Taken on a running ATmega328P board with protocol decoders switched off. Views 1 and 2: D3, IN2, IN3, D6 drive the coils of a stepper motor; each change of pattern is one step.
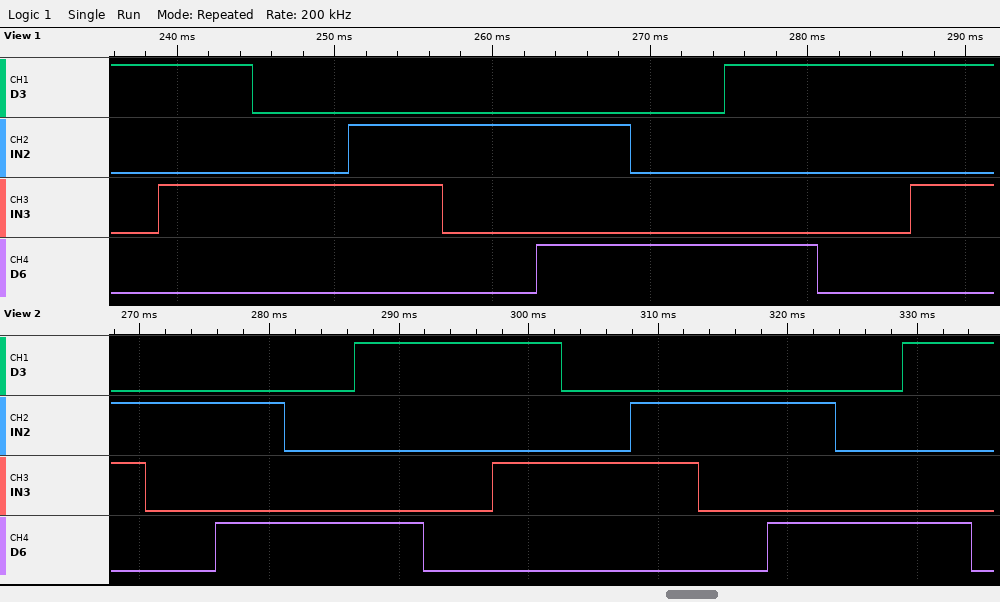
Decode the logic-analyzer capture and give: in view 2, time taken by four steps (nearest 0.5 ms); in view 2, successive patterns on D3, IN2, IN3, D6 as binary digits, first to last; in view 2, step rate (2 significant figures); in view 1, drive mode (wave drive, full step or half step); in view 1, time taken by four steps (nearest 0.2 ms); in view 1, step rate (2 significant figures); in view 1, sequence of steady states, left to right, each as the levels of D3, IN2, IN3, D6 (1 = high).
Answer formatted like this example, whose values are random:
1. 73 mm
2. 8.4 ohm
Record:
1. 21.5 ms
2. 0110 0100 0101 0001 1001 1000 1010 0010 0110 0100 0101 0001 1001 1000
3. 190 steps/s
4. half step
5. 24.0 ms
6. 170 steps/s
7. 1000 1010 0010 0110 0100 0101 0001 1001 1000 1010
